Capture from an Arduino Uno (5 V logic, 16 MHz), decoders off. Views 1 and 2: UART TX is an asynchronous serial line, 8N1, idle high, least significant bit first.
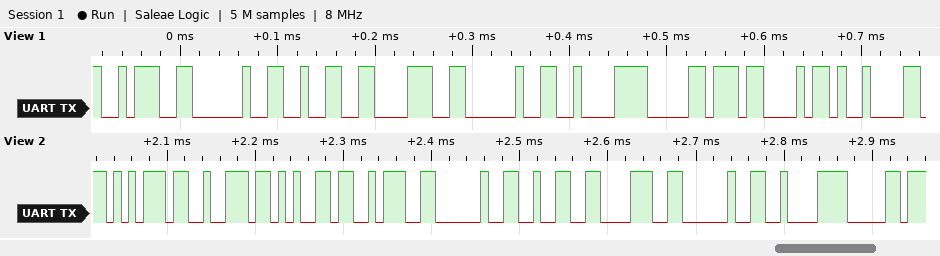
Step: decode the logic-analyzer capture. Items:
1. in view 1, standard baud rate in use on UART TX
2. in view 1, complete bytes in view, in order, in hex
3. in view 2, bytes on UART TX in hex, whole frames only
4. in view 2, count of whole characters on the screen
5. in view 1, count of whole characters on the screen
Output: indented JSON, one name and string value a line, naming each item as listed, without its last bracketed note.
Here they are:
{
  "in view 1, standard baud rate in use on UART TX": "115200 baud",
  "in view 1, complete bytes in view, in order, in hex": "3A 20 32 38 20 C2 B0 43 09",
  "in view 2, bytes on UART TX in hex, whole frames only": "0x75 0x72 0x65 0x3A 0x20 0x32 0x38 0x20 0xC2 0xB0",
  "in view 2, count of whole characters on the screen": "10",
  "in view 1, count of whole characters on the screen": "9"
}
